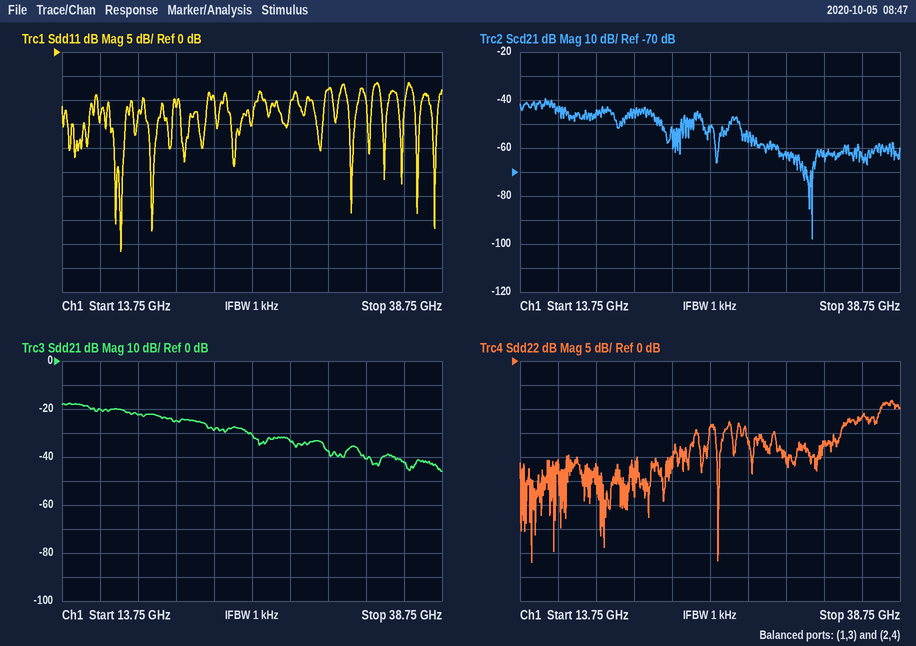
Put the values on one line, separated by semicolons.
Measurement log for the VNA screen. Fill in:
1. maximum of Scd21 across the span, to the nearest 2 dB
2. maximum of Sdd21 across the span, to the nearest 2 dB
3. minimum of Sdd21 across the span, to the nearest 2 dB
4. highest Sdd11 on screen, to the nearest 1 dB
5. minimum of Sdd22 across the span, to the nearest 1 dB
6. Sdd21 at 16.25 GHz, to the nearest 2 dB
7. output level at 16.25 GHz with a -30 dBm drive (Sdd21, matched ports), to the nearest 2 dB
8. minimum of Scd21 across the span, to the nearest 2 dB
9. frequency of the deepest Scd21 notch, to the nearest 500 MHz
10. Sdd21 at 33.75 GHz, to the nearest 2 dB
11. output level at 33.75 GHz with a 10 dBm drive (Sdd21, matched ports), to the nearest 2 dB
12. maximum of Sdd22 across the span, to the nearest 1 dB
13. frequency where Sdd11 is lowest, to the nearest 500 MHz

-40 dB; -18 dB; -46 dB; -6 dB; -42 dB; -20 dB; -50 dBm; -98 dB; 33.0 GHz; -40 dB; -30 dBm; -8 dB; 17.5 GHz
